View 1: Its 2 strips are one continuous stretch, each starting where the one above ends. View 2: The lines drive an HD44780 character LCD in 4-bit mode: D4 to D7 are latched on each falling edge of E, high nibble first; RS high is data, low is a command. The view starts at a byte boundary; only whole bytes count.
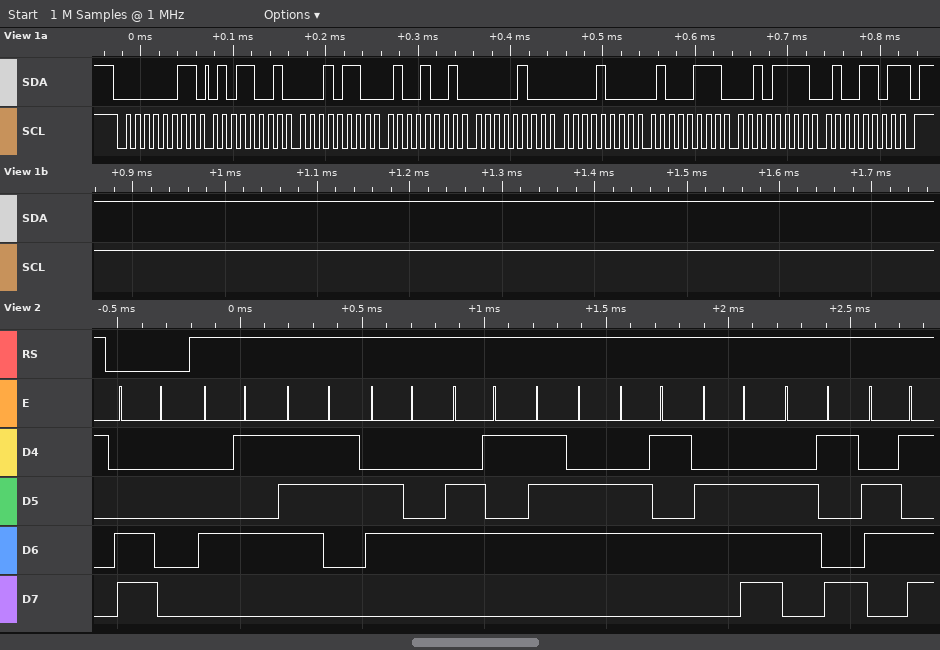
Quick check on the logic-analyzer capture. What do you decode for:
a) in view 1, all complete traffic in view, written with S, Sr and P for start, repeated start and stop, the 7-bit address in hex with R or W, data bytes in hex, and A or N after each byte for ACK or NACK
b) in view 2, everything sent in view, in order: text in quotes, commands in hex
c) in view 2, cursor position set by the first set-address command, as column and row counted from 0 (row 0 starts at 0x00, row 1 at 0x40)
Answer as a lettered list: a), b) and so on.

a) S 01R A 59 A 16 A 49 A 04 A 08 A 47 A 2F A 4D N P
b) 0xC0 "Esdevenim"
c) column 0, row 1
